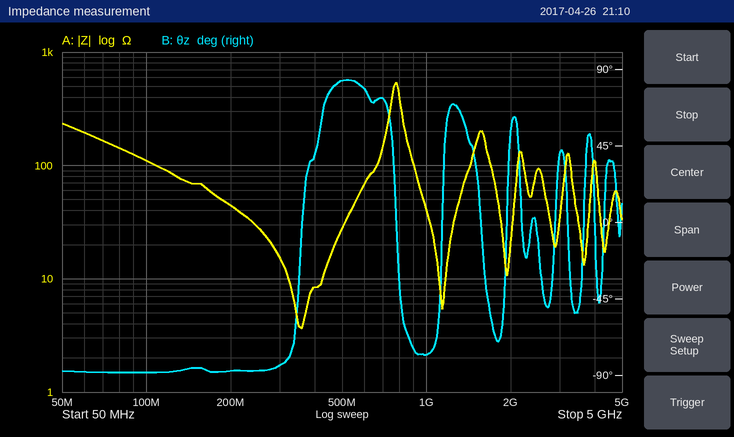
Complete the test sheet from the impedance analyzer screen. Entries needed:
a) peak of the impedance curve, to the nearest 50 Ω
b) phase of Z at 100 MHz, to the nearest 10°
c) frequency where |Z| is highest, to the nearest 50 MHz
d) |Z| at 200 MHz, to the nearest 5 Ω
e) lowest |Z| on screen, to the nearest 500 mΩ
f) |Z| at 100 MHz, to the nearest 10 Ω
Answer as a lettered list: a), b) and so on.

a) 550 Ω
b) -90°
c) 800 MHz
d) 45 Ω
e) 3.5 Ω
f) 110 Ω
